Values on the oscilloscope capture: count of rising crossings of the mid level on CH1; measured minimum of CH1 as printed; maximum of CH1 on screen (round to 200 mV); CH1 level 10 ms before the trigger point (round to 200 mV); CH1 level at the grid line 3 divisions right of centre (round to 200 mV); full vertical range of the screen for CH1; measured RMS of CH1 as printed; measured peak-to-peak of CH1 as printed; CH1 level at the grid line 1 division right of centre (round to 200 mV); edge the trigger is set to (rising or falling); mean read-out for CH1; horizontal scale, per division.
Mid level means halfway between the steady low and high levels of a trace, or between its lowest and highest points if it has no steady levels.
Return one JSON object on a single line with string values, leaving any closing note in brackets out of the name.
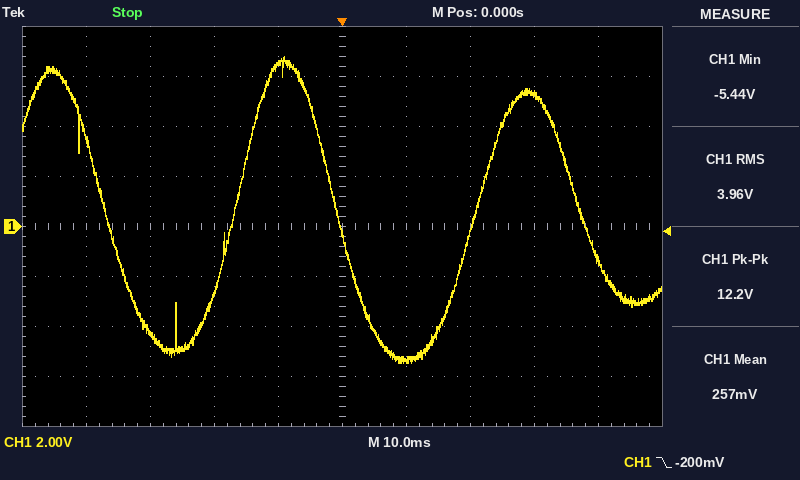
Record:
{"count of rising crossings of the mid level on CH1": "2", "measured minimum of CH1 as printed": "-5.44 V", "maximum of CH1 on screen": "6.8 V", "CH1 level 10 ms before the trigger point": "6.4 V", "CH1 level at the grid line 3 divisions right of centre": "5.2 V", "full vertical range of the screen for CH1": "16 V", "measured RMS of CH1 as printed": "3.96 V", "measured peak-to-peak of CH1 as printed": "12.2 V", "CH1 level at the grid line 1 division right of centre": "-5.4 V", "edge the trigger is set to": "falling", "mean read-out for CH1": "257 mV", "horizontal scale, per division": "10 ms"}
